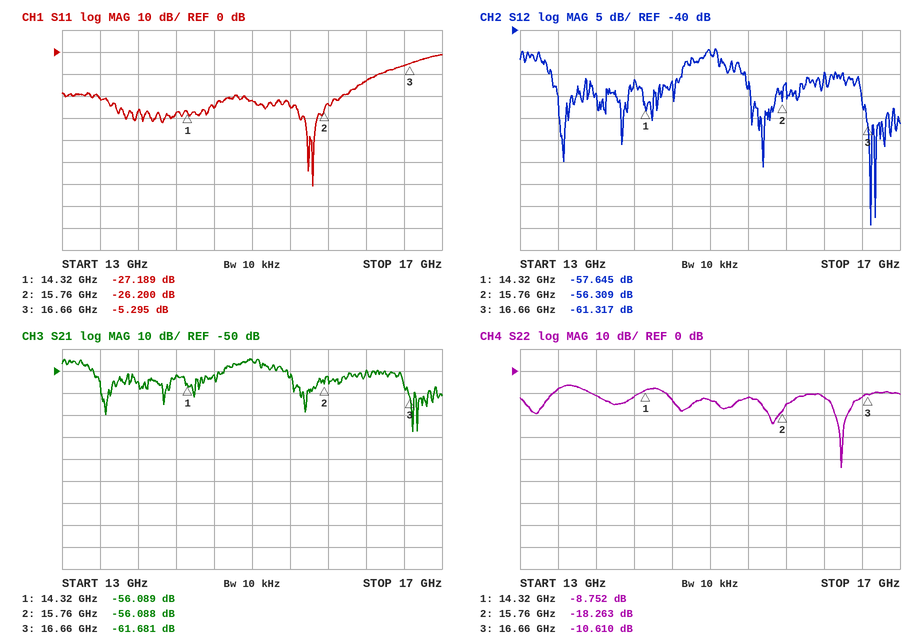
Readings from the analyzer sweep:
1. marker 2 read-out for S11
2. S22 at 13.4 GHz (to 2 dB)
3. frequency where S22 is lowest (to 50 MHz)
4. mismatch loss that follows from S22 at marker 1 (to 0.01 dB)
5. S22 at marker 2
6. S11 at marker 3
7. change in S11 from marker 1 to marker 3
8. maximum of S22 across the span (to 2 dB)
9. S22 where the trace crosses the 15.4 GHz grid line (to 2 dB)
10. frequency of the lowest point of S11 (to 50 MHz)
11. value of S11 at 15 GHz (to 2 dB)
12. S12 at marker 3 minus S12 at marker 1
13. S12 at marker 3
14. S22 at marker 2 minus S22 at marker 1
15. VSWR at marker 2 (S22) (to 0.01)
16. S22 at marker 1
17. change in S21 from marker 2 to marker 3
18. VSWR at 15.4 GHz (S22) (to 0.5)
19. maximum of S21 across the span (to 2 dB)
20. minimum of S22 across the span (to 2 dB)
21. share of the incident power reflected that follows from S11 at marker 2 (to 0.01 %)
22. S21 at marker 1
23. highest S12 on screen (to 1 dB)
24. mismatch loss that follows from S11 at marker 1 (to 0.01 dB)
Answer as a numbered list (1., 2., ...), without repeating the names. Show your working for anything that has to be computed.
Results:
1. -26.200 dB
2. -8 dB
3. 16.40 GHz
4. −10 log10(1 − 10^(-8.752/10)) ≈ 0.62 dB
5. -18.263 dB
6. -5.295 dB
7. -5.295 − (-27.189) = 21.894 dB
8. -6 dB
9. -12 dB
10. 15.65 GHz
11. -22 dB
12. -61.317 − (-57.645) = -3.672 dB
13. -61.317 dB
14. -18.263 − (-8.752) = -9.511 dB
15. (1 + 0.1221)/(1 − 0.1221) ≈ 1.28
16. -8.752 dB
17. -61.681 − (-56.088) = -5.593 dB
18. |Γ| = 10^(-12/20) = 0.2512; VSWR = (1 + 0.2512)/(1 − 0.2512) ≈ 1.67, so 1.5 to the nearest 0.5
19. -44 dB
20. -44 dB
21. 10^(-26.2/10) ≈ 0.24 %
22. -56.089 dB
23. -44 dB
24. −10 log10(1 − 10^(-27.189/10)) ≈ 0.01 dB
